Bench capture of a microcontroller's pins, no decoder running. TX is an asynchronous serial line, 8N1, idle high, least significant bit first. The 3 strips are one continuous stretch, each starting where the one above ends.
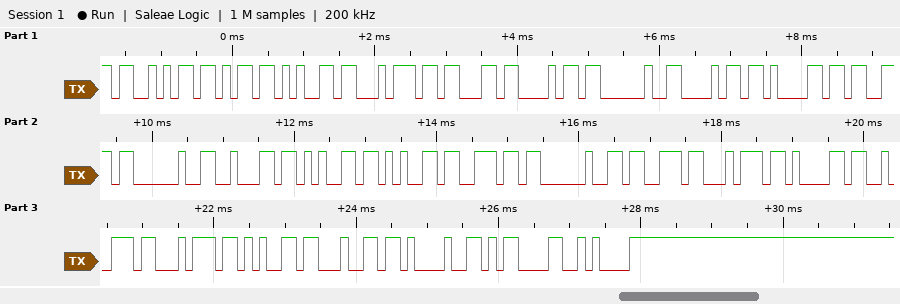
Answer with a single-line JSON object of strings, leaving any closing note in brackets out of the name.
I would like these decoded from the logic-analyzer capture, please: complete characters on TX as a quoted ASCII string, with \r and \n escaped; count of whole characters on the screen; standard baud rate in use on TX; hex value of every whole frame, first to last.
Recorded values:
{"complete characters on TX as a quoted ASCII string, with \\r and \\n escaped": "\"Sketch has been started!\\r\\n\"", "count of whole characters on the screen": "26", "standard baud rate in use on TX": "9600 baud", "hex value of every whole frame, first to last": "53 6B 65 74 63 68 20 68 61 73 20 62 65 65 6E 20 73 74 61 72 74 65 64 21 0D 0A"}
